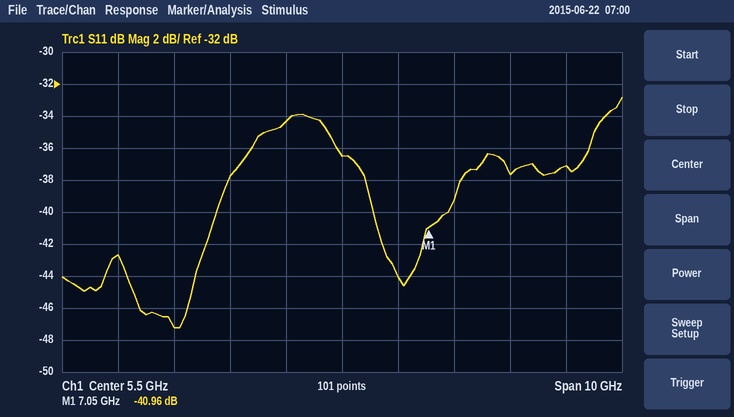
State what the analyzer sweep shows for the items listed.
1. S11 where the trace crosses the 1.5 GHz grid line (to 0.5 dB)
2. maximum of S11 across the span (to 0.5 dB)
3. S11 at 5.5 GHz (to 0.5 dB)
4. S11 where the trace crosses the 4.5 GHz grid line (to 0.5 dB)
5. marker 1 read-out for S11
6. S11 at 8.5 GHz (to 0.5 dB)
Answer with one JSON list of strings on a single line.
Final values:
["-42.5 dB", "-33.0 dB", "-36.5 dB", "-34.5 dB", "-40.96 dB", "-37.5 dB"]
